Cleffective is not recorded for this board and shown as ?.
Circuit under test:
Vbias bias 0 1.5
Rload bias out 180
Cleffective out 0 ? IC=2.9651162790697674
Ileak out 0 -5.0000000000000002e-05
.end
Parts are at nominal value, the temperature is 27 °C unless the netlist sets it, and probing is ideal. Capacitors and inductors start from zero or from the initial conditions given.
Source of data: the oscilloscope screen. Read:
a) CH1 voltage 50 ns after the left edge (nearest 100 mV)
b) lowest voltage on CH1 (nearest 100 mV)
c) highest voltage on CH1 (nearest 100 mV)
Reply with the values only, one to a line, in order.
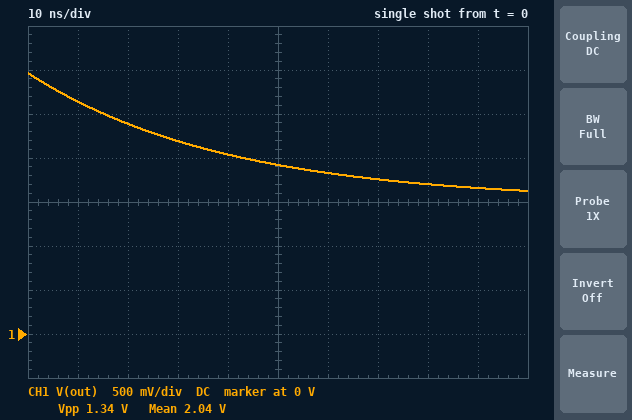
1.9 V
1.6 V
3.0 V
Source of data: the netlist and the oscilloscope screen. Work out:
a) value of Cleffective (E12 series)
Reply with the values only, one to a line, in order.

220 pF
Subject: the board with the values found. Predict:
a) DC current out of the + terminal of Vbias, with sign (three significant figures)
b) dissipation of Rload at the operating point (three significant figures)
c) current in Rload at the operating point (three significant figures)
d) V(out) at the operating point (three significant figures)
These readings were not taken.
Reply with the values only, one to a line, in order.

-50.0 µA
450 nW
50.0 µA
1.51 V
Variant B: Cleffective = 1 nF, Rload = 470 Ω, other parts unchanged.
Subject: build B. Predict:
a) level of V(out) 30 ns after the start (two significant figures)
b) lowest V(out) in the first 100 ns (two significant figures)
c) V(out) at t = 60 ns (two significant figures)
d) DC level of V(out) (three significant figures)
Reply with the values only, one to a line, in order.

2.9 V
2.7 V
2.8 V
1.52 V
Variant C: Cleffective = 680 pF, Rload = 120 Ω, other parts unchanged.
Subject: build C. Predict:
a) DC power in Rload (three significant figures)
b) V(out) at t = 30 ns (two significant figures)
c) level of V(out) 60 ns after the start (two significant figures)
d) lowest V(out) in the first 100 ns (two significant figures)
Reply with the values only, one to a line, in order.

300 nW
2.5 V
2.2 V
1.9 V
